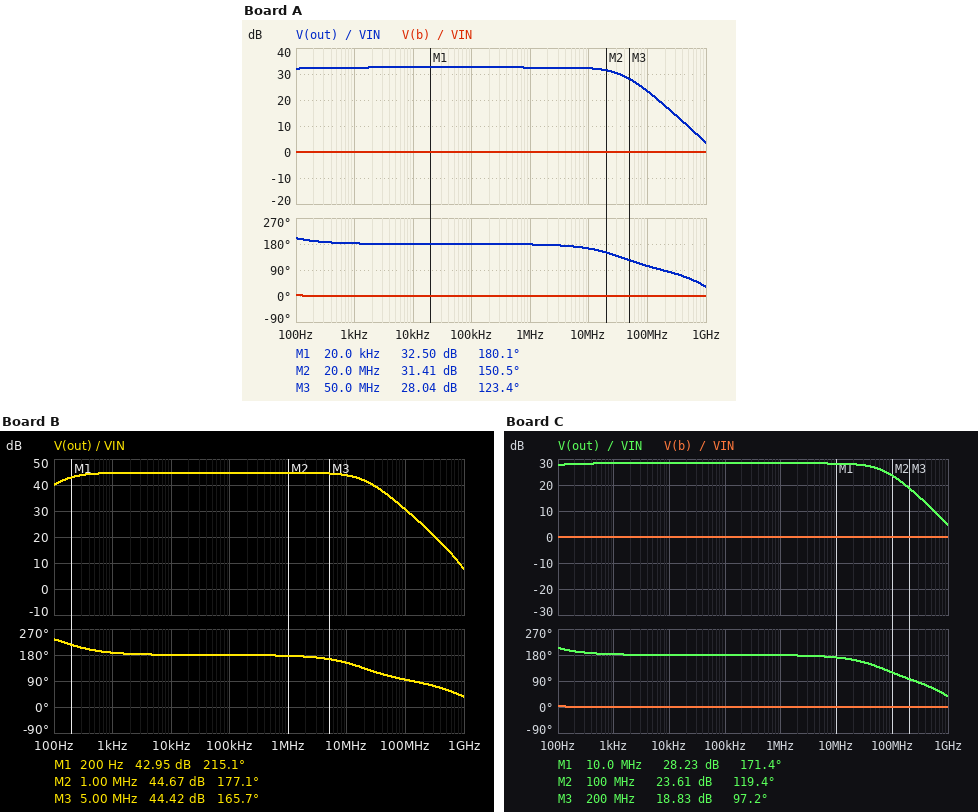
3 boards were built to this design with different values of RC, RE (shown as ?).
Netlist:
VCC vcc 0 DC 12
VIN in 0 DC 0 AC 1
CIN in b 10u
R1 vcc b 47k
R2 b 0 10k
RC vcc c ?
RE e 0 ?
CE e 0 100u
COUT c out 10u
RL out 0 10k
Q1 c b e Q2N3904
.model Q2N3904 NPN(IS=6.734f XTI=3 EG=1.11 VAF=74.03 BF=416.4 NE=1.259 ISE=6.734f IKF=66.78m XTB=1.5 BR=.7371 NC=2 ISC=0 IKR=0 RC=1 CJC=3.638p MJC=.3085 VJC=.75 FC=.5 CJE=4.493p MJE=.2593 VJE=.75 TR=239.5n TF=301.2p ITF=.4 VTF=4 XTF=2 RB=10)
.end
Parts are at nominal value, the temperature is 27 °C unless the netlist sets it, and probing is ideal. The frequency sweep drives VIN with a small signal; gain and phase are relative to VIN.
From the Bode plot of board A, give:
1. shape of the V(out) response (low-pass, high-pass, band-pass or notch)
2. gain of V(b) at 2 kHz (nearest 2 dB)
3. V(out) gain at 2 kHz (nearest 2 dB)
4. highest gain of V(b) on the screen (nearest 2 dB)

low-pass
0 dB
32 dB
0 dB
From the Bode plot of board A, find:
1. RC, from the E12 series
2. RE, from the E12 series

2.7 kΩ
2.7 kΩ
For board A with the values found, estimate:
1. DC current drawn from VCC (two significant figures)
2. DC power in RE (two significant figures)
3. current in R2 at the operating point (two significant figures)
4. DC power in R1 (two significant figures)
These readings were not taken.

740 µA
750 µW
210 µA
2.1 mW
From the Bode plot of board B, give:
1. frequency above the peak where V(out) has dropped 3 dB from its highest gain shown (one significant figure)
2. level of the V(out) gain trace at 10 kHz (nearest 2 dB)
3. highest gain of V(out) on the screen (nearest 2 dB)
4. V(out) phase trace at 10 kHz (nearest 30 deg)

20 MHz
44 dB
44 dB
180 deg
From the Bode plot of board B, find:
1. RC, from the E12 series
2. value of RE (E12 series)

2.7 kΩ
560 Ω
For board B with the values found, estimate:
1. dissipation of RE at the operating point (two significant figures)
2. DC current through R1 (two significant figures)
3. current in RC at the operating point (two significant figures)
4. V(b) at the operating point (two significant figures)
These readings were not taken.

3.0 mW
210 µA
2.3 mA
2.0 V
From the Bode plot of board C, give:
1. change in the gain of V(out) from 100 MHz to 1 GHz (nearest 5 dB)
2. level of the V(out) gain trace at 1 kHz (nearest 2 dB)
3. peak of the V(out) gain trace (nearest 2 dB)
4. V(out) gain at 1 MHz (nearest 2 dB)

-20 dB
28 dB
28 dB
28 dB
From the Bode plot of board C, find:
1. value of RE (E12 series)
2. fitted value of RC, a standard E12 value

2.2 kΩ
1.2 kΩ
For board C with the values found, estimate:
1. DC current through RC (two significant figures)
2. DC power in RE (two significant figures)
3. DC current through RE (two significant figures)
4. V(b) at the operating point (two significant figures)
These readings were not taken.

640 µA
910 µW
640 µA
2.1 V
